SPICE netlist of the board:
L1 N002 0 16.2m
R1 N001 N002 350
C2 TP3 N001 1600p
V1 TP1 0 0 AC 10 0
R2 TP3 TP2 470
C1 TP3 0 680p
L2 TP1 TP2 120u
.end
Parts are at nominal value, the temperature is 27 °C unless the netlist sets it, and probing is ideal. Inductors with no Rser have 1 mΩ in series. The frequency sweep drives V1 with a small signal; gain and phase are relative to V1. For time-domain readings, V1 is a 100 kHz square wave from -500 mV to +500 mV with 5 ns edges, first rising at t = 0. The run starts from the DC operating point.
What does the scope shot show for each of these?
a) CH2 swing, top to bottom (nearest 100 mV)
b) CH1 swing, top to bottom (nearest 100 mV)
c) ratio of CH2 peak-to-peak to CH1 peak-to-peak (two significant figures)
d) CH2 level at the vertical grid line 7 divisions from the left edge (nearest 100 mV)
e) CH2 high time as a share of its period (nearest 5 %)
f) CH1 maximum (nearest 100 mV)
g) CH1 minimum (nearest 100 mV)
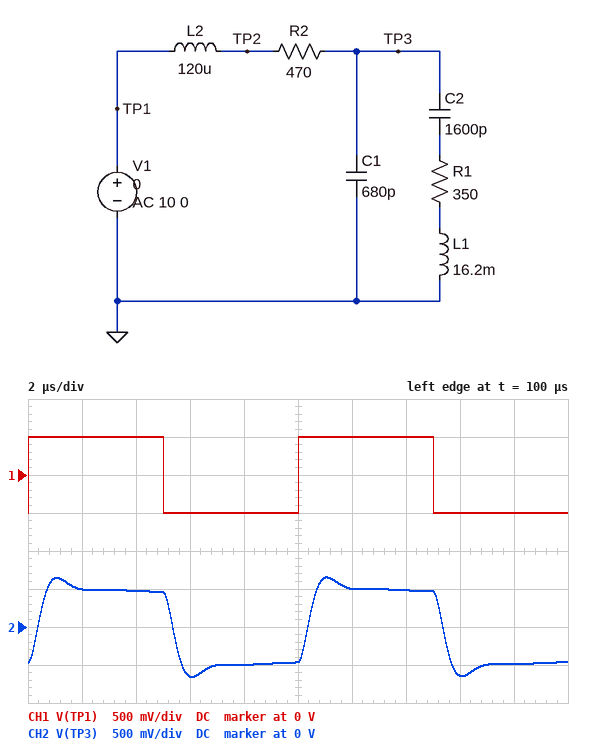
1.3 V
1.0 V
1.3
500 mV
50 %
500 mV
-500 mV
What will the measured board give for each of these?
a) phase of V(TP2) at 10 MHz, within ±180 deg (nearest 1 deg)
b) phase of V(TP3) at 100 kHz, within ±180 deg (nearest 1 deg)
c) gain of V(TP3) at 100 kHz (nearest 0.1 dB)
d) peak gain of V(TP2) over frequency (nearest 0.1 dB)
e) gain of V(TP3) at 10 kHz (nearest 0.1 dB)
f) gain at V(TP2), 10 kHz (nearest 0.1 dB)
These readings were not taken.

-89 deg
-9 deg
0.1 dB
2.9 dB
0 dB
0 dB
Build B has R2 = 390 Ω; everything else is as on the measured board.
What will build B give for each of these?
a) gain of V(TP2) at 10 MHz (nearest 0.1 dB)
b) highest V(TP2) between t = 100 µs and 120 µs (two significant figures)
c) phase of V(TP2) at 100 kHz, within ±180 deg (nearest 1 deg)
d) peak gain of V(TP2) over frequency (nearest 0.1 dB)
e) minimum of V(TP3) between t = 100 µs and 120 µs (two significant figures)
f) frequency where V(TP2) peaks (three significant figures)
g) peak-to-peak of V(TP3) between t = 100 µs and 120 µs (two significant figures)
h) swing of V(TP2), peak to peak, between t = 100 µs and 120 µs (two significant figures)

-25.7 dB
820 mV
0 deg
3.7 dB
-720 mV
486 kHz
1.4 V
1.6 V
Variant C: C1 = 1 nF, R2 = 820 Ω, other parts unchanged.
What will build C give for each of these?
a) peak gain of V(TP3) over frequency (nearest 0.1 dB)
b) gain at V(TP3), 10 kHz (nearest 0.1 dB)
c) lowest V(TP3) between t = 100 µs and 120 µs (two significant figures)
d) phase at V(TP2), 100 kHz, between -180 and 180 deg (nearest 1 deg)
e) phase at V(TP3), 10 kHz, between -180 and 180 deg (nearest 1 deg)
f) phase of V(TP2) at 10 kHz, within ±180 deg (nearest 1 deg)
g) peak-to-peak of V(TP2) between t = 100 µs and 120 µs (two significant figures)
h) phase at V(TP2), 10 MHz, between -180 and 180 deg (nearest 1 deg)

0 dB
-0.1 dB
-510 mV
-1 deg
-8 deg
0 deg
1.2 V
-85 deg
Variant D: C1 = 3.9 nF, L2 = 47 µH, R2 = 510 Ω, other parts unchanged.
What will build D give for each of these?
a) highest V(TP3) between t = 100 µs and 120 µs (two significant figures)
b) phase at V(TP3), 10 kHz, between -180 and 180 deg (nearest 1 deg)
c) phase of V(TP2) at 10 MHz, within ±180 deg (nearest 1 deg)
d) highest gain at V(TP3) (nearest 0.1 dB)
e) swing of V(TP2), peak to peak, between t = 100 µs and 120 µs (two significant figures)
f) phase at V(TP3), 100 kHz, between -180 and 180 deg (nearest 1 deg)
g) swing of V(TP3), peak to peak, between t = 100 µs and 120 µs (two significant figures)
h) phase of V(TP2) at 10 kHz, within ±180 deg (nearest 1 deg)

440 mV
-10 deg
-81 deg
0 dB
1.1 V
-52 deg
870 mV
0 deg
